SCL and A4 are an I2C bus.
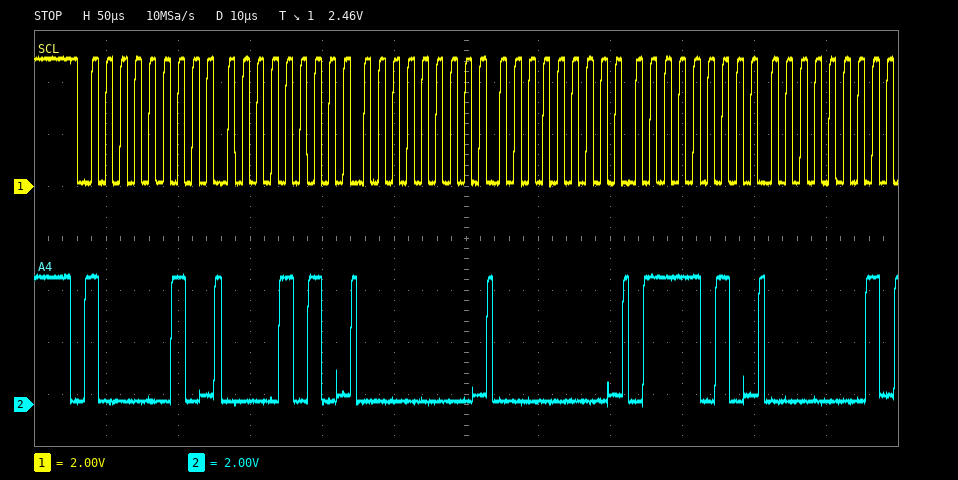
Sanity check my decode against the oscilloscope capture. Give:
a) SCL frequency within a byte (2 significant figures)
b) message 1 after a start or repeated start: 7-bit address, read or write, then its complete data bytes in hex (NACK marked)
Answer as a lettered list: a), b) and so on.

a) 100 kHz
b) 0x41 write: 0A 00 00 7A 01
